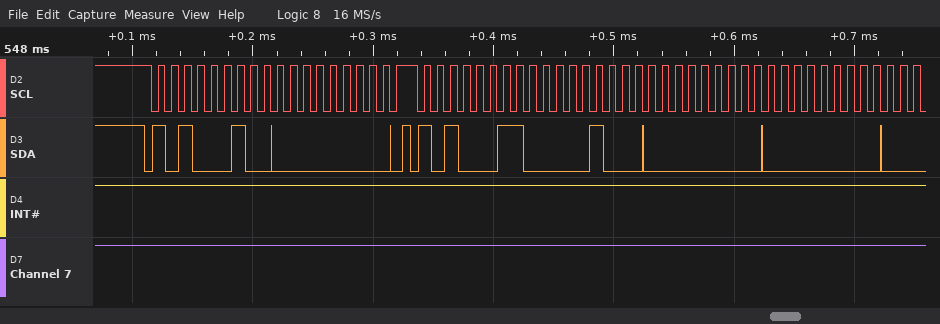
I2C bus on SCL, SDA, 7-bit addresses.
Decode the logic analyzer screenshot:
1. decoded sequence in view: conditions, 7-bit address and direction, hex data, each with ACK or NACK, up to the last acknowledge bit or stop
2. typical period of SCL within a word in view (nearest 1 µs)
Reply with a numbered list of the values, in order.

1. start, address 51 write ACK, 00 ACK, stop, start, address 51 read ACK, 08 ACK, 00 ACK, 00 ACK
2. 11 µs
